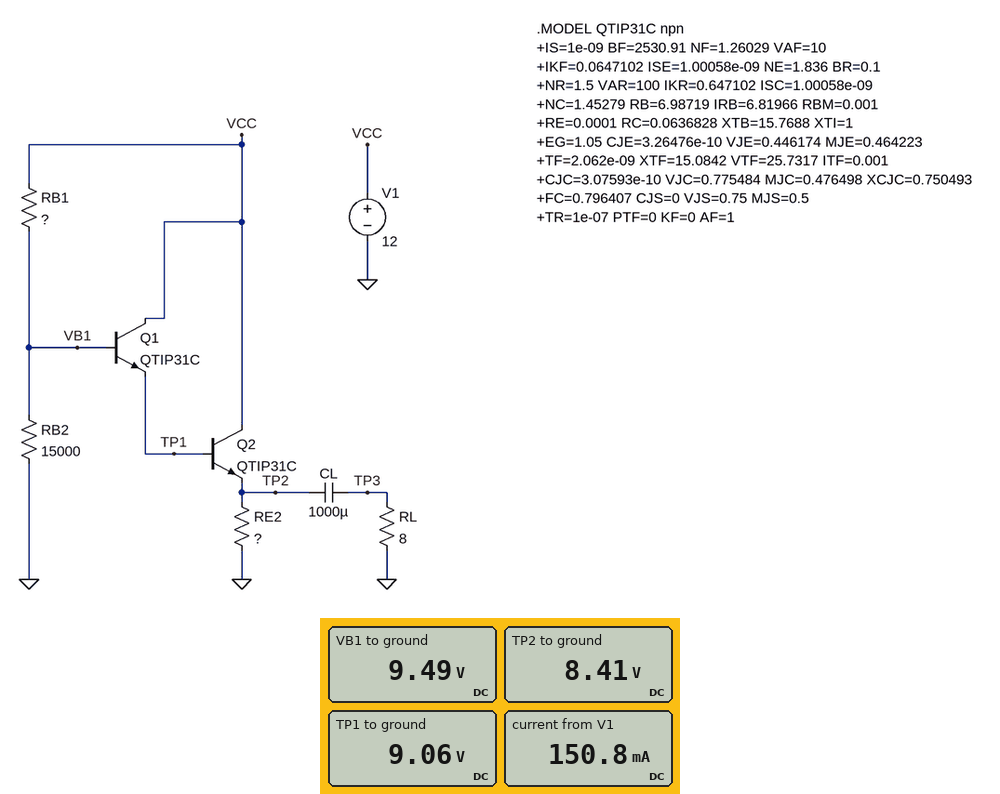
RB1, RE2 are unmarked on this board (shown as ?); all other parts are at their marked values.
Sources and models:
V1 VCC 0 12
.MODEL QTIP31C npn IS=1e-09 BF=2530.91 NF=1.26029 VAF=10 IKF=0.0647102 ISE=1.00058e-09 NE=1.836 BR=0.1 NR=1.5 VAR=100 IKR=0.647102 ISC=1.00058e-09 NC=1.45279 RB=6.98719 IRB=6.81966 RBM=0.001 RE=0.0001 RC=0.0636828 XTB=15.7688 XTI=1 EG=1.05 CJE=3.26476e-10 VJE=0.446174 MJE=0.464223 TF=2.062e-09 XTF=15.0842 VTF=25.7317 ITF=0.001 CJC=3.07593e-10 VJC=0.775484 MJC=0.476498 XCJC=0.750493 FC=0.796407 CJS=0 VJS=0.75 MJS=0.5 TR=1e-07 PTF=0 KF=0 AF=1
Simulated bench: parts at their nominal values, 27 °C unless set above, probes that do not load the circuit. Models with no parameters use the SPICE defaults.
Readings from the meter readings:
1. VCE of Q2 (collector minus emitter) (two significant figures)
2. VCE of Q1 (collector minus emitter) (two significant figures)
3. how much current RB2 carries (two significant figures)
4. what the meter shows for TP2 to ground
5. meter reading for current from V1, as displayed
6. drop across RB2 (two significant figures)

3.6 V
2.9 V
630 µA
8.41 V
150.8 mA
9.5 V
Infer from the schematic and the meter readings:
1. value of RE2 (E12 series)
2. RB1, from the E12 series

56 Ω
3.9 kΩ
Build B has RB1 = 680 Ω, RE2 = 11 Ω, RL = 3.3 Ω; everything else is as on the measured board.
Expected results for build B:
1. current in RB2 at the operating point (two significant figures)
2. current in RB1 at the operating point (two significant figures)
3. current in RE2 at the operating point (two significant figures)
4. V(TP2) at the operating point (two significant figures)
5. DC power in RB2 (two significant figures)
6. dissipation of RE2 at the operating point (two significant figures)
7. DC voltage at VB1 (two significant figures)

760 µA
850 µA
910 mA
10 V
8.7 mW
9.2 W
11 V
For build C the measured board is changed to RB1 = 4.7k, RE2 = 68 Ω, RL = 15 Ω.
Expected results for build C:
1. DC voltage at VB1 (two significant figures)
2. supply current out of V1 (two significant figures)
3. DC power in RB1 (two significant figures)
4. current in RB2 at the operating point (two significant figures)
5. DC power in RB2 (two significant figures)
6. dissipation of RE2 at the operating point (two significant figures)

9.1 V
120 mA
1.8 mW
610 µA
5.5 mW
950 mW
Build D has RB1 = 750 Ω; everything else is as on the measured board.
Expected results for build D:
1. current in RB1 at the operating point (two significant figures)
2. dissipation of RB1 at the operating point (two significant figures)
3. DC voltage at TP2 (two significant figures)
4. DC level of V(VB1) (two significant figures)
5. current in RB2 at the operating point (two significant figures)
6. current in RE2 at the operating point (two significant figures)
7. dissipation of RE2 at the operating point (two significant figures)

780 µA
450 µW
10 V
11 V
760 µA
180 mA
1.9 W
